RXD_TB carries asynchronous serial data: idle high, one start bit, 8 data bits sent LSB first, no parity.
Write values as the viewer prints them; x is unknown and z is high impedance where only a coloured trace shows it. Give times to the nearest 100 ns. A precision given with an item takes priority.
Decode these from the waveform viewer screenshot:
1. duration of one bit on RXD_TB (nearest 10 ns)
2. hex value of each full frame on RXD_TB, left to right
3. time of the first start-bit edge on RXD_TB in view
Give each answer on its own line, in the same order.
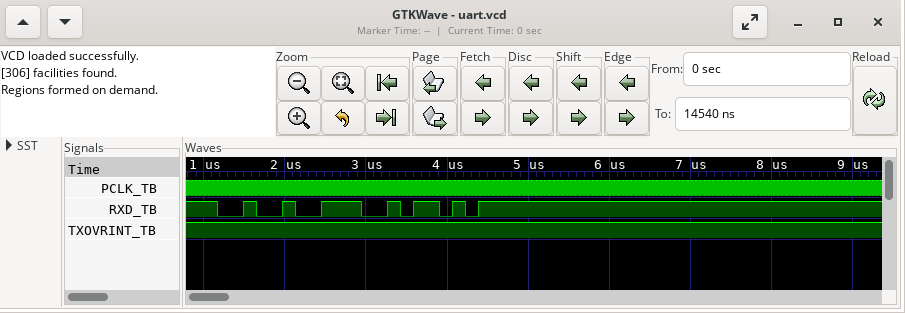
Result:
160 ns
92, 5A
1200 ns
